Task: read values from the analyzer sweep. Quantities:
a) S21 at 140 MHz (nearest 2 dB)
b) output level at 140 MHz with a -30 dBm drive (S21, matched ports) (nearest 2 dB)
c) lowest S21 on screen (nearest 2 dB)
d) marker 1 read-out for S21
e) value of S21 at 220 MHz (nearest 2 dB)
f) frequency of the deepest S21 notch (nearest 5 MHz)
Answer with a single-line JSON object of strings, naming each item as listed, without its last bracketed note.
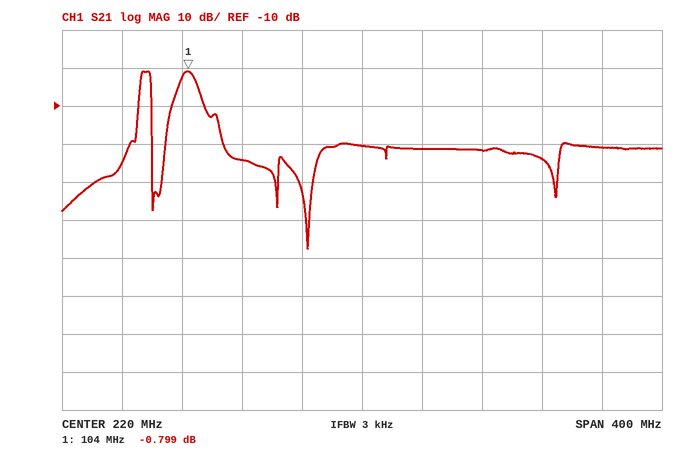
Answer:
{"S21 at 140 MHz": "-24 dB", "output level at 140 MHz with a -30 dBm drive (S21, matched ports)": "-54 dBm", "lowest S21 on screen": "-48 dB", "marker 1 read-out for S21": "-0.799 dB", "value of S21 at 220 MHz": "-20 dB", "frequency of the deepest S21 notch": "185 MHz"}
